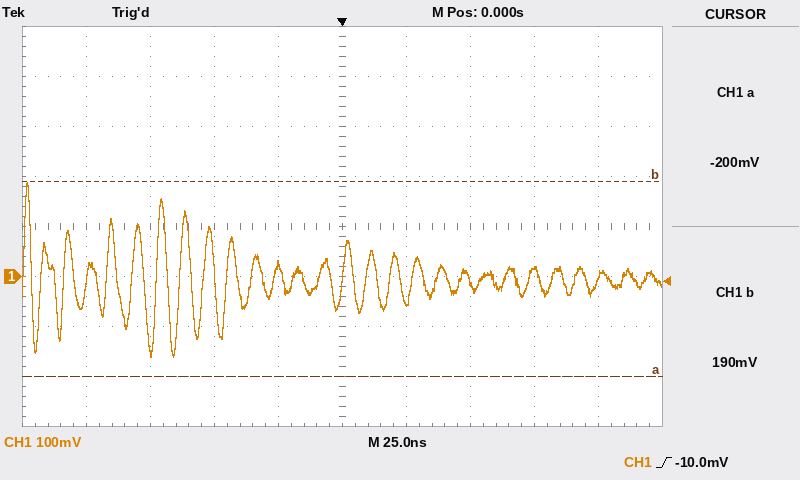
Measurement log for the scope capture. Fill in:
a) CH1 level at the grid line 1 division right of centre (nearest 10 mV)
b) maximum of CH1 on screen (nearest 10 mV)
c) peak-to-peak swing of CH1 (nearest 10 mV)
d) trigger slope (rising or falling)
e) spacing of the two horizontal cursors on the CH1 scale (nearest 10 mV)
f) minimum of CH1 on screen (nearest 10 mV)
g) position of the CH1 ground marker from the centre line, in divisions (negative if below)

-50 mV
190 mV
350 mV
rising
390 mV
-160 mV
-1.0 div
